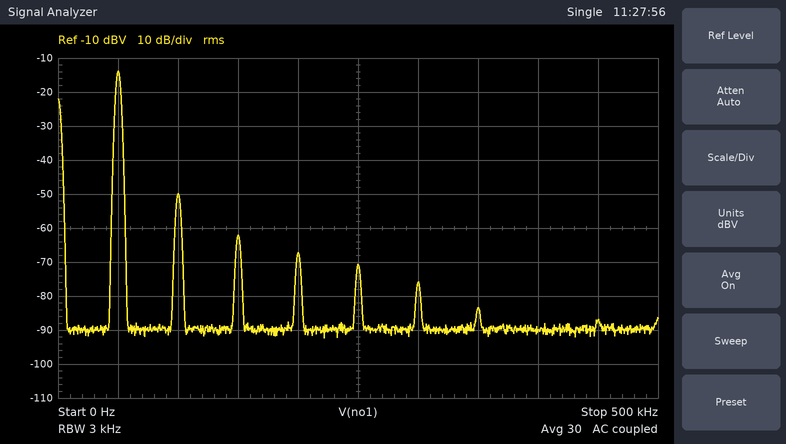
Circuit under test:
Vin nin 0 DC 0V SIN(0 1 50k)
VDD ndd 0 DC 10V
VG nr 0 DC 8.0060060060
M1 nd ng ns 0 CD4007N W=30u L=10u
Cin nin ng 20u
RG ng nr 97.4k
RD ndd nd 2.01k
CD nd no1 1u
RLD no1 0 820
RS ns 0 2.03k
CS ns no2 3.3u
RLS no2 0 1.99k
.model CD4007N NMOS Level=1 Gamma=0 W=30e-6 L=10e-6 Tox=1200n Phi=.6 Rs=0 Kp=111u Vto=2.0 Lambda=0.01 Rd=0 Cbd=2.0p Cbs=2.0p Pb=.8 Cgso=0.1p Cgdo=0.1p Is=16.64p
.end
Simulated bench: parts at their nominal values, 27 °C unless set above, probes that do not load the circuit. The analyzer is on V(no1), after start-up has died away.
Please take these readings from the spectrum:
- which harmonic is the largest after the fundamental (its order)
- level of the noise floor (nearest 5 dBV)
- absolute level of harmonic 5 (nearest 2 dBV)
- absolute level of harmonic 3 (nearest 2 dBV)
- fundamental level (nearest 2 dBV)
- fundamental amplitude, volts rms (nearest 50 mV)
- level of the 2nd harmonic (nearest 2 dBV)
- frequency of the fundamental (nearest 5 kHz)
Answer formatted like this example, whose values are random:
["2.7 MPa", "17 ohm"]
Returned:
["2", "-90 dBV", "-70 dBV", "-62 dBV", "-14 dBV", "200 mV", "-50 dBV", "50 kHz"]
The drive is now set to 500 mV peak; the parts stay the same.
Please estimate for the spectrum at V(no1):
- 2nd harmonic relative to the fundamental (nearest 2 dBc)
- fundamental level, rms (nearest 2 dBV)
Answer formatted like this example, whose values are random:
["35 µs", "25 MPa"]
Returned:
["-40 dBc", "-20 dBV"]
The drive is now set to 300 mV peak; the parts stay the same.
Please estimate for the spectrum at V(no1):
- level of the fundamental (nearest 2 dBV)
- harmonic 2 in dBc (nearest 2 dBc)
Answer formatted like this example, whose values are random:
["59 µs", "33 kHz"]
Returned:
["-24 dBV", "-44 dBc"]
